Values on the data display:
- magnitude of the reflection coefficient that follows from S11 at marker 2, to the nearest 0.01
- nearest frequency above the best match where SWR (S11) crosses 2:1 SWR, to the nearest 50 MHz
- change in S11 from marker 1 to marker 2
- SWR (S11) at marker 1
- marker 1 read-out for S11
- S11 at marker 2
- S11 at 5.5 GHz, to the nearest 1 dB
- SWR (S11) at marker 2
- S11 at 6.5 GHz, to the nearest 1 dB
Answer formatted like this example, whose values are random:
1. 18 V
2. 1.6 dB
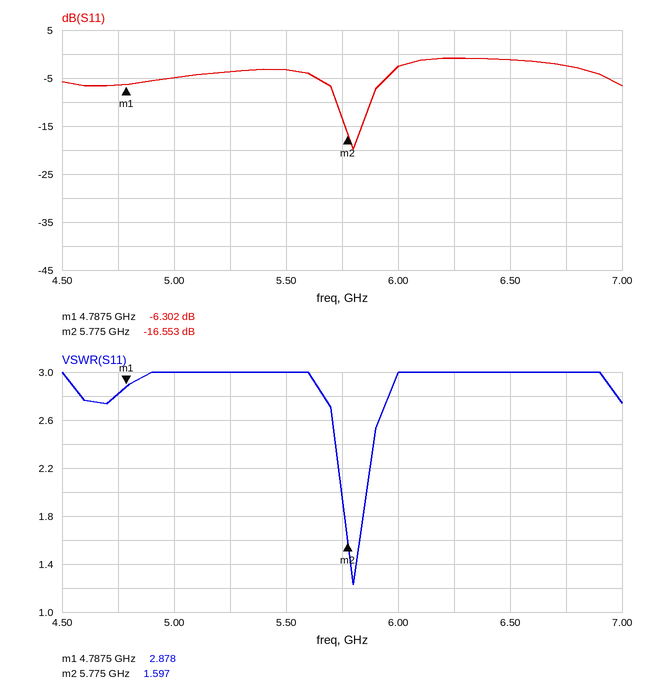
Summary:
1. 0.15
2. 5.85 GHz
3. -10.251 dB
4. 2.878
5. -6.302 dB
6. -16.553 dB
7. -3 dB
8. 1.597
9. -1 dB
